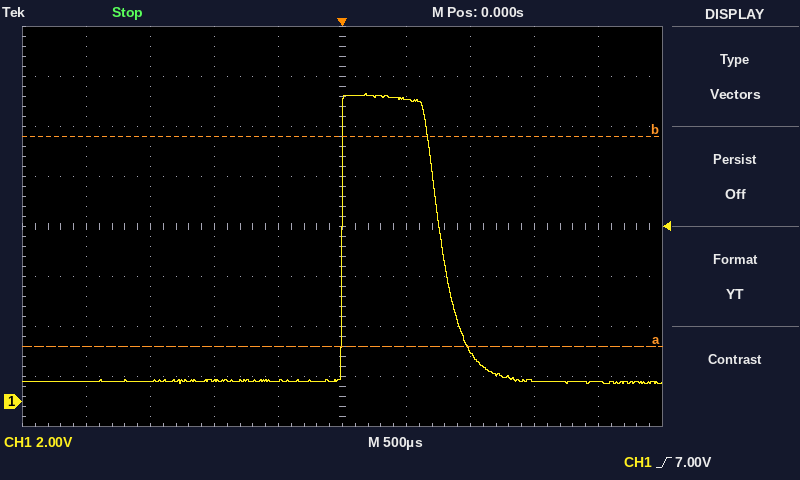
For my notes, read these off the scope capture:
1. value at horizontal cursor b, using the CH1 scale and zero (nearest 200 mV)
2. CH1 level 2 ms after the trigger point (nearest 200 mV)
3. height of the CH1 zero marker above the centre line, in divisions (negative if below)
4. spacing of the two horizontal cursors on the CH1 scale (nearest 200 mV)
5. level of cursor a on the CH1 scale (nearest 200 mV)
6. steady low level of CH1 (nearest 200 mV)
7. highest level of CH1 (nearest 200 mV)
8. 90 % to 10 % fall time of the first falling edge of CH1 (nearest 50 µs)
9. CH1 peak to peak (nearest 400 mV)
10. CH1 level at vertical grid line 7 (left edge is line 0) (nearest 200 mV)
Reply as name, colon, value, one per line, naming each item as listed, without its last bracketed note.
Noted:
value at horizontal cursor b, using the CH1 scale and zero: 10.6 V
CH1 level 2 ms after the trigger point: 800 mV
height of the CH1 zero marker above the centre line, in divisions: -3.5 div
spacing of the two horizontal cursors on the CH1 scale: 8.4 V
level of cursor a on the CH1 scale: 2.2 V
steady low level of CH1: 800 mV
highest level of CH1: 12.4 V
90 % to 10 % fall time of the first falling edge of CH1: 350 µs
CH1 peak to peak: 11.6 V
CH1 level at vertical grid line 7 (left edge is line 0): 2.0 V
